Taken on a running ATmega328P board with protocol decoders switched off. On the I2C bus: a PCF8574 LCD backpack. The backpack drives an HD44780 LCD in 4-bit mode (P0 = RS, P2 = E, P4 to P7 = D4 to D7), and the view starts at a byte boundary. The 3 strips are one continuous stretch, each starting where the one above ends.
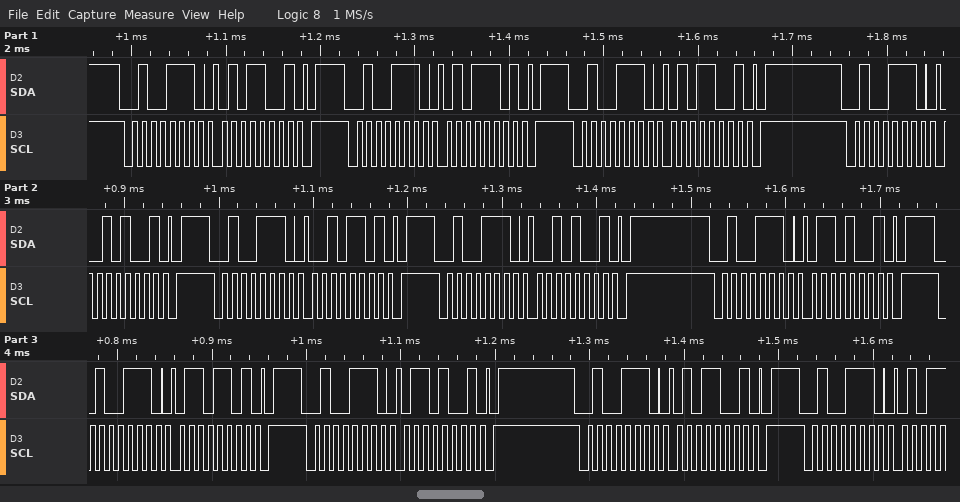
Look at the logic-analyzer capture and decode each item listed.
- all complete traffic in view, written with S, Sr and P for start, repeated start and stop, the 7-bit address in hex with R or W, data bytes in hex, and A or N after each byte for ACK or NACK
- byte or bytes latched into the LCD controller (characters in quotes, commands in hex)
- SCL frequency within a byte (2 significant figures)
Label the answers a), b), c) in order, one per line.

a) S 27W A 59 A P S 27W A 5D A P S 27W A 59 A P S 27W A 29 A P S 27W A 2D A P S 27W A 29 A P S 27W A 69 A P S 27W A 6D A P S 27W A 69 A P S 27W A 59 A P S 27W A
b) 'R'
c) 100 kHz
